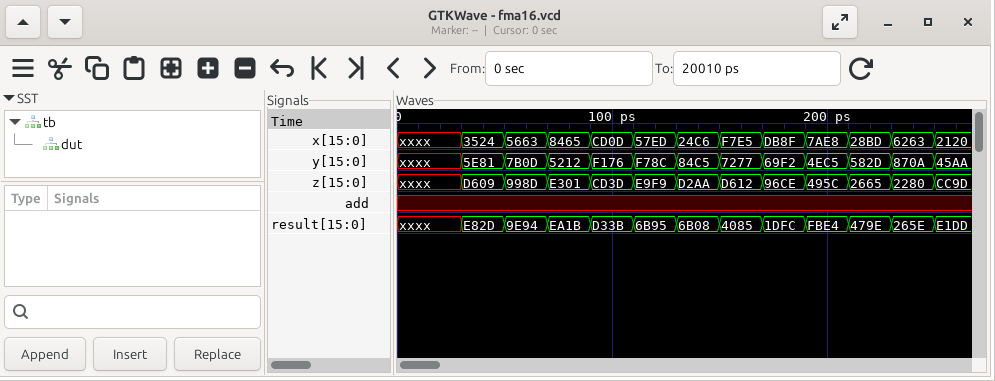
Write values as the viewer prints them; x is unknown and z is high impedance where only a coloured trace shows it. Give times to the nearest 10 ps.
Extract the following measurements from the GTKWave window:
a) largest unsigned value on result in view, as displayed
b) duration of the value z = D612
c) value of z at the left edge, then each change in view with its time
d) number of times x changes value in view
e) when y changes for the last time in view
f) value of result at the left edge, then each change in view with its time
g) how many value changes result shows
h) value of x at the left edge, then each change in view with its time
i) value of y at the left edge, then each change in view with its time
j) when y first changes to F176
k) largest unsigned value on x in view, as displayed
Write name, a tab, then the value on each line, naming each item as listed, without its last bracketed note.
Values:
largest unsigned value on result in view, as displayed	FBE4
duration of the value z = D612	20 ps
value of z at the left edge, then each change in view with its time	xxxx, D609 at 30 ps, 998D at 50 ps, E301 at 70 ps, CD3D at 90 ps, E9F9 at 110 ps, D2AA at 130 ps, D612 at 150 ps, 96CE at 170 ps, 495C at 190 ps, 2665 at 210 ps, 2280 at 230 ps, CC9D at 250 ps
number of times x changes value in view	12
when y changes for the last time in view	250 ps
value of result at the left edge, then each change in view with its time	xxxx, E82D at 30 ps, 9E94 at 50 ps, EA1B at 70 ps, D33B at 90 ps, 6B95 at 110 ps, 6B08 at 130 ps, 4085 at 150 ps, 1DFC at 170 ps, FBE4 at 190 ps, 479E at 210 ps, 265E at 230 ps, E1DD at 250 ps
how many value changes result shows	12
value of x at the left edge, then each change in view with its time	xxxx, 3524 at 30 ps, 5663 at 50 ps, 8465 at 70 ps, CD0D at 90 ps, 57ED at 110 ps, 24C6 at 130 ps, F7E5 at 150 ps, DB8F at 170 ps, 7AE8 at 190 ps, 28BD at 210 ps, 6263 at 230 ps, 2120 at 250 ps
value of y at the left edge, then each change in view with its time	xxxx, 5E81 at 30 ps, 7B0D at 50 ps, 5212 at 70 ps, F176 at 90 ps, F78C at 110 ps, 84C5 at 130 ps, 7277 at 150 ps, 69F2 at 170 ps, 4EC5 at 190 ps, 582D at 210 ps, 870A at 230 ps, 45AA at 250 ps
when y first changes to F176	90 ps
largest unsigned value on x in view, as displayed	F7E5
